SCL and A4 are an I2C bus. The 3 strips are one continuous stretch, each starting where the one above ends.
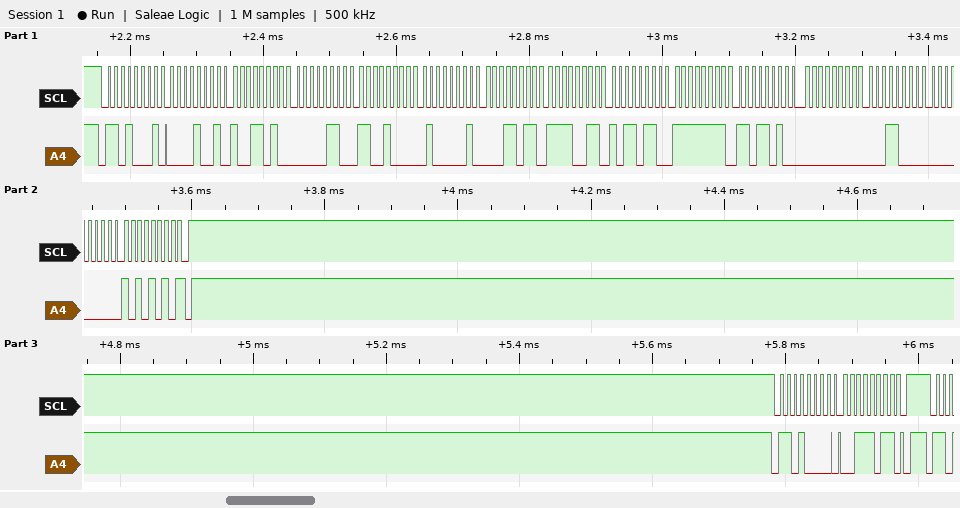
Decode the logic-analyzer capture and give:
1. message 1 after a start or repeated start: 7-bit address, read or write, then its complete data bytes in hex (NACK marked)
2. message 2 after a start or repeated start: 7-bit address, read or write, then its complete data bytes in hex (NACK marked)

0x68 read: 09 9A 06 C8 41 1B F3 B6 FF DA 00 18 00 AA NACK
0x68 write: 3B
